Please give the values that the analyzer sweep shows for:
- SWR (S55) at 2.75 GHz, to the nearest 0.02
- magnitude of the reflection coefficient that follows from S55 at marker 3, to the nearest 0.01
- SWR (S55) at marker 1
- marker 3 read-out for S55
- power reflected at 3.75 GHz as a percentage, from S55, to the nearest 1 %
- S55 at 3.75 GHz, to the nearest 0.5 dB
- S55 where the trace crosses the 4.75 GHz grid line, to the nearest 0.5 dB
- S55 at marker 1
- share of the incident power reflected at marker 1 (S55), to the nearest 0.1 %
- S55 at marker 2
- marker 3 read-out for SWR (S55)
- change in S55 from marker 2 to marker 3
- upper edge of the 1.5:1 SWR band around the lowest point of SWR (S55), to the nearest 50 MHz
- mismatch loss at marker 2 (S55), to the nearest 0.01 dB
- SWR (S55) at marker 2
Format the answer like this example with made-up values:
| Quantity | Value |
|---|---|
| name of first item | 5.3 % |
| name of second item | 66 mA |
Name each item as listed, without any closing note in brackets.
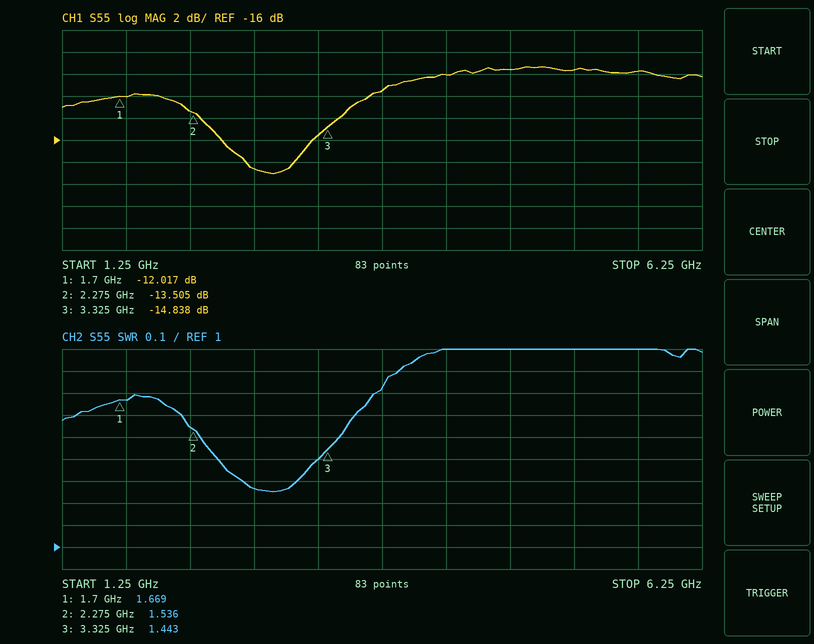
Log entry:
| Quantity | Value |
|---|---|
| SWR (S55) at 2.75 GHz, to the nearest 0.02 | 1.26 |
| magnitude of the reflection coefficient that follows from S55 at marker 3, to the nearest 0.01 | 0.18 |
| SWR (S55) at marker 1 | 1.669 |
| marker 3 read-out for S55 | -14.838 dB |
| power reflected at 3.75 GHz as a percentage, from S55, to the nearest 1 % | 7 % |
| S55 at 3.75 GHz, to the nearest 0.5 dB | -11.5 dB |
| S55 where the trace crosses the 4.75 GHz grid line, to the nearest 0.5 dB | -9.5 dB |
| S55 at marker 1 | -12.017 dB |
| share of the incident power reflected at marker 1 (S55), to the nearest 0.1 % | 6.3 % |
| S55 at marker 2 | -13.505 dB |
| marker 3 read-out for SWR | 1.443 |
| change in S55 from marker 2 to marker 3 | -1.333 dB |
| upper edge of the 1.5:1 SWR band around the lowest point of SWR (S55), to the nearest 50 MHz | 3.40 GHz |
| mismatch loss at marker 2 (S55), to the nearest 0.01 dB | 0.20 dB |
| SWR (S55) at marker 2 | 1.536 |
